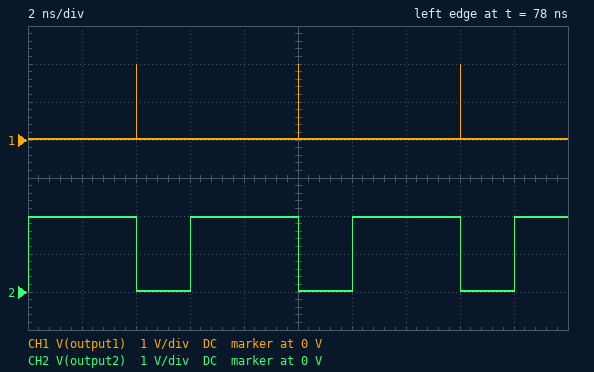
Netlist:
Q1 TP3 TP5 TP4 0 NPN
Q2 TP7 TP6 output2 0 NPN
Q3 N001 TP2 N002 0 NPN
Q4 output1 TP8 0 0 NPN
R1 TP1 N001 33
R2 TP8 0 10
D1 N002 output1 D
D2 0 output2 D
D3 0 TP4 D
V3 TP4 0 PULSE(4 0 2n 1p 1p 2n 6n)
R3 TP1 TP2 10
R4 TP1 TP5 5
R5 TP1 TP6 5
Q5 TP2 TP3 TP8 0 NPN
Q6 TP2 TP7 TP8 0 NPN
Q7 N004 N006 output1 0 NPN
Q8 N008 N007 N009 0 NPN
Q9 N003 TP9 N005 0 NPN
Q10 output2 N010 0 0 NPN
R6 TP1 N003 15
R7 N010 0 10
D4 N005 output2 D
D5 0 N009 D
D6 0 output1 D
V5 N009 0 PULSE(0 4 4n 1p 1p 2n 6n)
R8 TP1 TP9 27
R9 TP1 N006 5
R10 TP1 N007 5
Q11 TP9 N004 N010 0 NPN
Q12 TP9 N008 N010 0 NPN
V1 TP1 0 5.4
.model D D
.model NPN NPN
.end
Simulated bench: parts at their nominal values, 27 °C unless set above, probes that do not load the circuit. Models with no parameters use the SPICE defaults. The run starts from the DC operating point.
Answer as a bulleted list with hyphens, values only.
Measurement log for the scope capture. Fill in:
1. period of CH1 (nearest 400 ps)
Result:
- 6.0 ns
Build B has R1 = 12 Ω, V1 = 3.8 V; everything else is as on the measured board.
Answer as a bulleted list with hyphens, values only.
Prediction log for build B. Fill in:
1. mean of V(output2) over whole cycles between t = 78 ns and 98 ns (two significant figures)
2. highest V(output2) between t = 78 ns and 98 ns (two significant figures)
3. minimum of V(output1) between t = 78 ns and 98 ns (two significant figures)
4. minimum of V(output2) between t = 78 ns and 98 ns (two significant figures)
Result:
- 1.3 V
- 1.9 V
- 26 mV
- 27 mV
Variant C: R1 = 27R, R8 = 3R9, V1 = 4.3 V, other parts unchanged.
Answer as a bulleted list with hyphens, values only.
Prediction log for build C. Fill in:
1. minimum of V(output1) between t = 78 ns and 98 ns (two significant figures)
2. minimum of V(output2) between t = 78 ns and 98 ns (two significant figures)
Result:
- 24 mV
- 23 mV
